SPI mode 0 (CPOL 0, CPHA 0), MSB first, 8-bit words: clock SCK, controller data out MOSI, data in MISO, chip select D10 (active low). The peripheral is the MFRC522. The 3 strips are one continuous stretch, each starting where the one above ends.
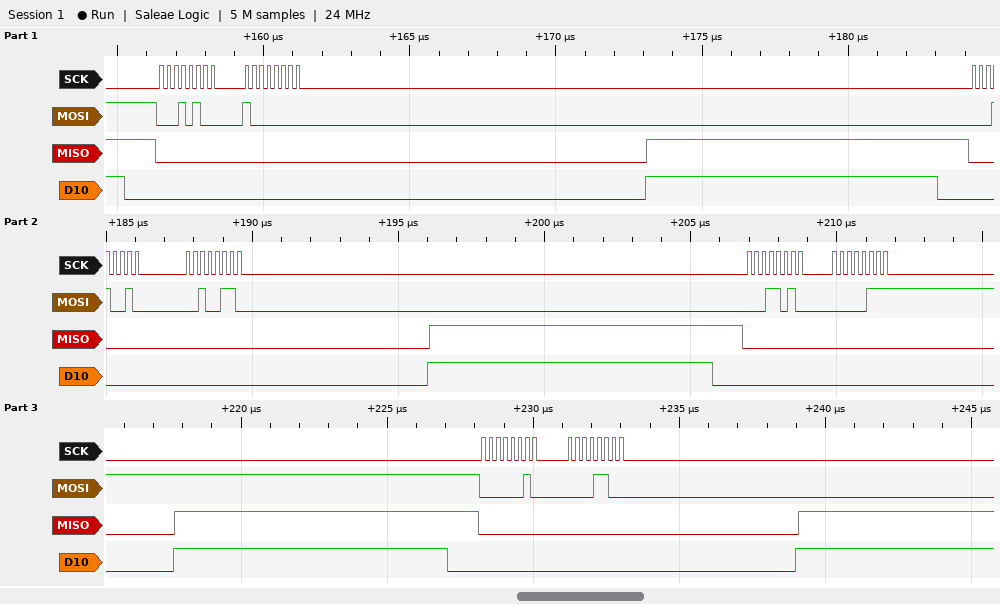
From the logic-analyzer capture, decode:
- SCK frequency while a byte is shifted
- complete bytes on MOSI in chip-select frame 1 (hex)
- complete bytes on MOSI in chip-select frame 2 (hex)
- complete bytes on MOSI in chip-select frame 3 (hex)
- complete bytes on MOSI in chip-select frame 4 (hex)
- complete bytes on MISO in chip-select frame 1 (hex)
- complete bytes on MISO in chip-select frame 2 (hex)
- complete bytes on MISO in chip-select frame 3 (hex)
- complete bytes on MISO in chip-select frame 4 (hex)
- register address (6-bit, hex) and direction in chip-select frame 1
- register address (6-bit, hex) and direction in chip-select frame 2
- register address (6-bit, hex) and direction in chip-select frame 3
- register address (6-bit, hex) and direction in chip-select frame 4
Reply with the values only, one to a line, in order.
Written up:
4 MHz
14 80
12 26
1A 07
02 0C
00 00
00 00
00 00
00 00
0x0A write
0x09 write
0x0D write
0x01 write
